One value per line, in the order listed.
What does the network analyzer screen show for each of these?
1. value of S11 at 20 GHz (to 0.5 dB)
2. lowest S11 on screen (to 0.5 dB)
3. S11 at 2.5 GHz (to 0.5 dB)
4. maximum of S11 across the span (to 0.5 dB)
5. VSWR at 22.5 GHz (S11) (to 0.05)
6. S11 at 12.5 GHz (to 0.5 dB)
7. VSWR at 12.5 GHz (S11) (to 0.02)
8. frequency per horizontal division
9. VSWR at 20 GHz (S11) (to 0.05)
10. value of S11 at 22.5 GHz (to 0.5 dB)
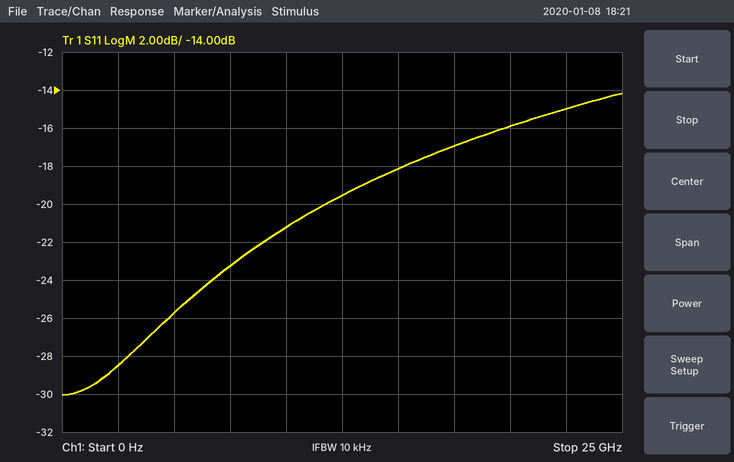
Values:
-16.0 dB
-30.0 dB
-28.5 dB
-14.0 dB
1.45
-19.5 dB
1.24
2.5 GHz
1.40
-15.0 dB
